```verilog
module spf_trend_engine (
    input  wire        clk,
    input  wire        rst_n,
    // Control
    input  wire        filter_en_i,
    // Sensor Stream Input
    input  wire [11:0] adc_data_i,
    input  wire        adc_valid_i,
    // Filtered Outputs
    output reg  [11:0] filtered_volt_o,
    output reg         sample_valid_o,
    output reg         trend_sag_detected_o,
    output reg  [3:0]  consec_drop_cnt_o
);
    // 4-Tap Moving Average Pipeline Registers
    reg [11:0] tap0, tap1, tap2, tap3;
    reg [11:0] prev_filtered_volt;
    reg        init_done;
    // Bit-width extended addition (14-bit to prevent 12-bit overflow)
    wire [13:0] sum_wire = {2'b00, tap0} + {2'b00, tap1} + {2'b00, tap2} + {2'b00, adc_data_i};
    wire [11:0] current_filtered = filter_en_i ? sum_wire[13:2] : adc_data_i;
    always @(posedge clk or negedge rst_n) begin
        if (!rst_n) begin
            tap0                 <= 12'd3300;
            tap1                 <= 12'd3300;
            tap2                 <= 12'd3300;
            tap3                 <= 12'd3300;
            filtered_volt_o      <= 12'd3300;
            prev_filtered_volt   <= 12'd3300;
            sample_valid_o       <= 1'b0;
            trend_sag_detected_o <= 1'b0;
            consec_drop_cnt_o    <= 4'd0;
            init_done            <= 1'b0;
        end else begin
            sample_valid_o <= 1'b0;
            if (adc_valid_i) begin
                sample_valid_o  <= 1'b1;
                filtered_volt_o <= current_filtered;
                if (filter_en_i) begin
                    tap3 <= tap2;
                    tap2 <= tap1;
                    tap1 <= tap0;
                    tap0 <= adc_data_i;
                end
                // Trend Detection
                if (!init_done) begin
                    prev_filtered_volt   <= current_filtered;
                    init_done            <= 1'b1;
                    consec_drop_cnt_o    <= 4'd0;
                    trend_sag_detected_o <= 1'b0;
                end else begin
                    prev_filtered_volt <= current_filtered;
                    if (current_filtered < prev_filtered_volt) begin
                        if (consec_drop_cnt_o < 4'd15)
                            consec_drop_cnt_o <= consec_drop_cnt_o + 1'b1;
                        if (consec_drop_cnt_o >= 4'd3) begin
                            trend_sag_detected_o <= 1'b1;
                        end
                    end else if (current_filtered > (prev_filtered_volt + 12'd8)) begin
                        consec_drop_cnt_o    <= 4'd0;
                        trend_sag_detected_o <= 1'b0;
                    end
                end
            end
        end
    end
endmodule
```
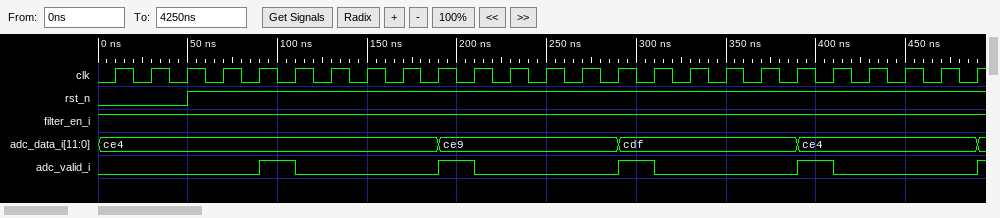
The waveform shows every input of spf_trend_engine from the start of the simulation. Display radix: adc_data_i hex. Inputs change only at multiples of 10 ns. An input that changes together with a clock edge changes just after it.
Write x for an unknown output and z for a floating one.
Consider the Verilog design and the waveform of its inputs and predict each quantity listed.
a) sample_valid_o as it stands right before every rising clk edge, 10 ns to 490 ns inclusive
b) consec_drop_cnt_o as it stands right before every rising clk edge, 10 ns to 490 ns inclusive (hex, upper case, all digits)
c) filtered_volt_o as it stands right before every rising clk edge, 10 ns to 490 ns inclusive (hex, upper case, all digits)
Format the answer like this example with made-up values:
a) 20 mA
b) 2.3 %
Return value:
a) 0 0 0 0 0 0 1 0 0 0 0 1 0 0 0 0 1 0 0 0 0 1 0 0 0
b) 0, 0, 0, 0, 0, 0, 0, 0, 0, 0, 0, 0, 0, 0, 0, 0, 1, 1, 1, 1, 1, 1, 1, 1, 1
c) CE4, CE4, CE4, CE4, CE4, CE4, CE4, CE4, CE4, CE4, CE4, CE5, CE5, CE5, CE5, CE5, CE4, CE4, CE4, CE4, CE4, CE4, CE4, CE4, CE4
